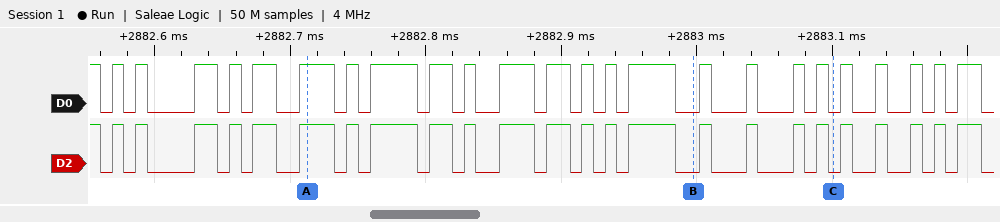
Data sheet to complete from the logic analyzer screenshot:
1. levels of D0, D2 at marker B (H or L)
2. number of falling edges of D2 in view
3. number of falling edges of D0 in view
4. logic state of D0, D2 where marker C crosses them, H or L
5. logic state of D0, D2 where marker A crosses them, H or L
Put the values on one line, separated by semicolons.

D0=L, D2=L; 25; 25; D0=L, D2=L; D0=H, D2=H
